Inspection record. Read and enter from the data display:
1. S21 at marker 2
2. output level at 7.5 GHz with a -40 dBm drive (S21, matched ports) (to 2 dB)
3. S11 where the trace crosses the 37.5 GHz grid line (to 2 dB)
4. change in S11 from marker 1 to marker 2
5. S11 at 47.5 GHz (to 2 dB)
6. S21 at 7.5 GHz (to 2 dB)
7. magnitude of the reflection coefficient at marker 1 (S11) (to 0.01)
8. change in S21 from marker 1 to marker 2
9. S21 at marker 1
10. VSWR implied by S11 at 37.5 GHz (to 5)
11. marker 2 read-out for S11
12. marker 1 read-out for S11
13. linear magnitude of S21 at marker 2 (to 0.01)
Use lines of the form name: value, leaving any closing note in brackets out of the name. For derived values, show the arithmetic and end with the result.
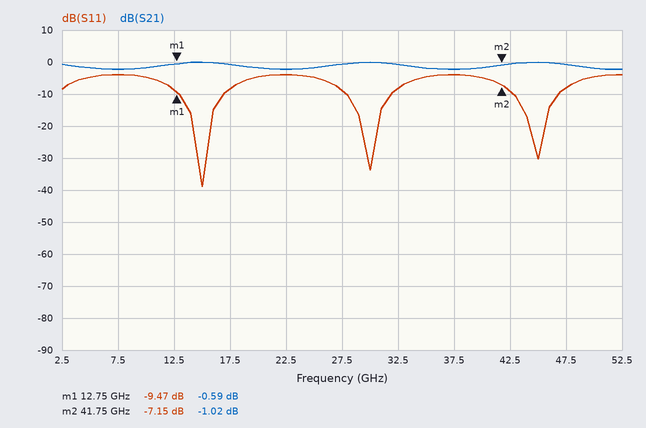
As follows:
S21 at marker 2: -1.02 dB
output level at 7.5 GHz with a -40 dBm drive (S21, matched ports): -40 dBm + (-2 dB) = -42 dBm
S11 where the trace crosses the 37.5 GHz grid line: -4 dB
change in S11 from marker 1 to marker 2: -7.15 − (-9.47) = 2.32 dB
S11 at 47.5 GHz: -8 dB
S21 at 7.5 GHz: -2 dB
magnitude of the reflection coefficient at marker 1 (S11): 10^(-9.47/20) ≈ 0.34
change in S21 from marker 1 to marker 2: -1.02 − (-0.59) = -0.43 dB
S21 at marker 1: -0.59 dB
VSWR implied by S11 at 37.5 GHz: |Γ| = 10^(-4/20) = 0.6310; VSWR = (1 + 0.6310)/(1 − 0.6310) ≈ 4.42, so 5 to the nearest 5
marker 2 read-out for S11: -7.15 dB
marker 1 read-out for S11: -9.47 dB
linear magnitude of S21 at marker 2: 10^(-1.02/20) ≈ 0.89
